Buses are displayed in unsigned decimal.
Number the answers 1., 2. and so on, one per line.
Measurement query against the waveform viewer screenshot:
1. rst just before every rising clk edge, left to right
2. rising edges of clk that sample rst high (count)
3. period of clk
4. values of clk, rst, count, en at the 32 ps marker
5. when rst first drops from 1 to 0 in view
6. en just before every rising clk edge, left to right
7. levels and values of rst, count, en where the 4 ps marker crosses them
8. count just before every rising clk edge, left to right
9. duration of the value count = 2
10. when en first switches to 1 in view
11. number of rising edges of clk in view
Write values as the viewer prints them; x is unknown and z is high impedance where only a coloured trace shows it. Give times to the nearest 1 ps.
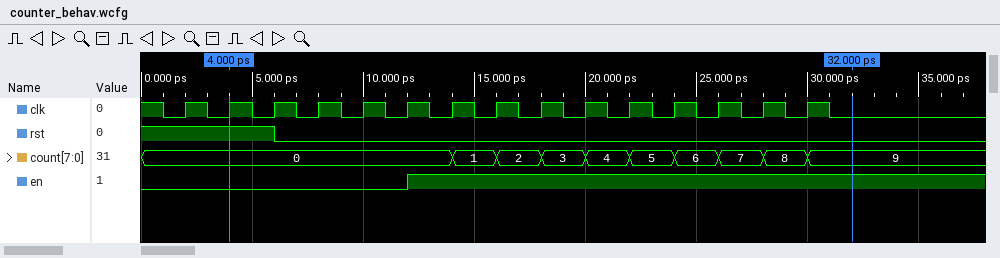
1. 1 1 1 0 0 0 0 0 0 0 0 0 0 0 0
2. 3
3. 2 ps
4. clk=0, rst=0, count=9, en=1
5. 6 ps
6. 0 0 0 0 0 0 1 1 1 1 1 1 1 1 1
7. rst=1, count=0, en=0
8. 0, 0, 0, 0, 0, 0, 0, 1, 2, 3, 4, 5, 6, 7, 8
9. 2 ps
10. 12 ps
11. 15
